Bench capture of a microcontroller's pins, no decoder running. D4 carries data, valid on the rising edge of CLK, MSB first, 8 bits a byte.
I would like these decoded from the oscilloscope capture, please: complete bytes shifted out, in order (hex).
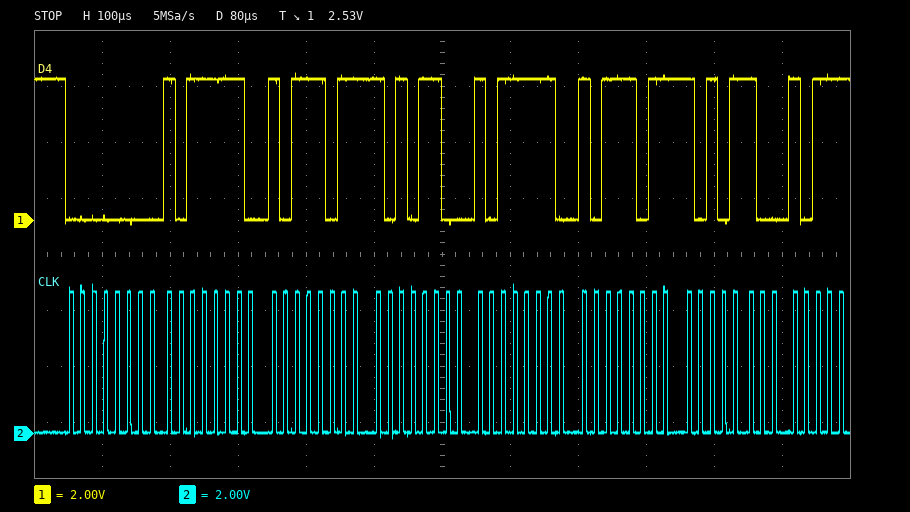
00 BE BB AC BE BB AC
